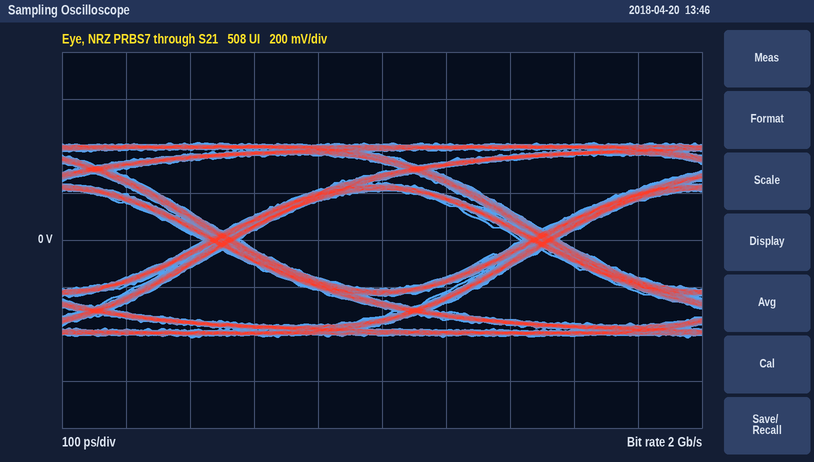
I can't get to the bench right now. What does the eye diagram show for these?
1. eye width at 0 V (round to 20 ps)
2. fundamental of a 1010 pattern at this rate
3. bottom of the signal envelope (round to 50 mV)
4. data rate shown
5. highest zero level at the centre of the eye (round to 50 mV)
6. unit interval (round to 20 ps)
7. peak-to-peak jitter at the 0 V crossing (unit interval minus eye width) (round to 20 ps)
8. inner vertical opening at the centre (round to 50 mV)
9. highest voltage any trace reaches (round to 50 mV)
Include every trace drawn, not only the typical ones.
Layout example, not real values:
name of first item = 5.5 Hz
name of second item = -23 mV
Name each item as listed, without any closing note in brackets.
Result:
eye width at 0 V = 440 ps
fundamental of a 1010 pattern at this rate = 1 GHz
bottom of the signal envelope = -400 mV
data rate shown = 2 Gb/s
highest zero level at the centre of the eye = -200 mV
unit interval = 500 ps
peak-to-peak jitter at the 0 V crossing (unit interval minus eye width) = 60 ps
inner vertical opening at the centre = 400 mV
highest voltage any trace reaches = 400 mV
